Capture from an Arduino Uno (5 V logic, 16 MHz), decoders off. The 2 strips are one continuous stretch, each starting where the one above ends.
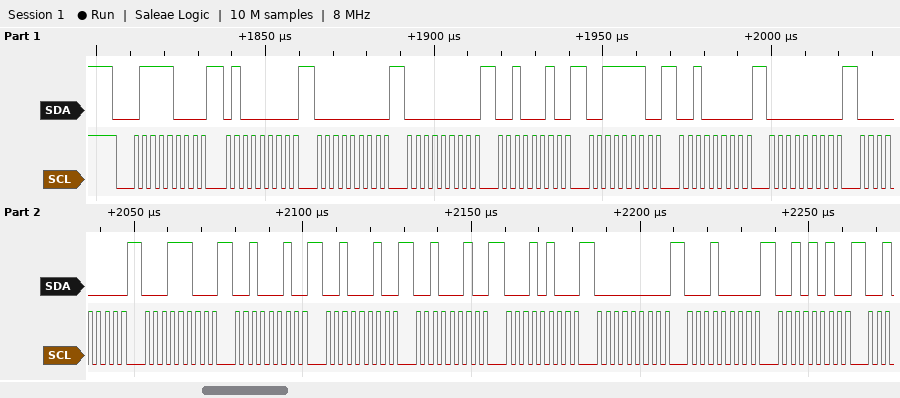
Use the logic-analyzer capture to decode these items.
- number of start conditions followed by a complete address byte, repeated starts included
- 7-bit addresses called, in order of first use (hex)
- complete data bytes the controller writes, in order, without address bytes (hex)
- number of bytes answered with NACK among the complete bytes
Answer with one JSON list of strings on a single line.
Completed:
["1", "0x3C", "40 00 00 22 3E 20 00 00 1C 22 22 22 14 00 10 2A", "0"]
